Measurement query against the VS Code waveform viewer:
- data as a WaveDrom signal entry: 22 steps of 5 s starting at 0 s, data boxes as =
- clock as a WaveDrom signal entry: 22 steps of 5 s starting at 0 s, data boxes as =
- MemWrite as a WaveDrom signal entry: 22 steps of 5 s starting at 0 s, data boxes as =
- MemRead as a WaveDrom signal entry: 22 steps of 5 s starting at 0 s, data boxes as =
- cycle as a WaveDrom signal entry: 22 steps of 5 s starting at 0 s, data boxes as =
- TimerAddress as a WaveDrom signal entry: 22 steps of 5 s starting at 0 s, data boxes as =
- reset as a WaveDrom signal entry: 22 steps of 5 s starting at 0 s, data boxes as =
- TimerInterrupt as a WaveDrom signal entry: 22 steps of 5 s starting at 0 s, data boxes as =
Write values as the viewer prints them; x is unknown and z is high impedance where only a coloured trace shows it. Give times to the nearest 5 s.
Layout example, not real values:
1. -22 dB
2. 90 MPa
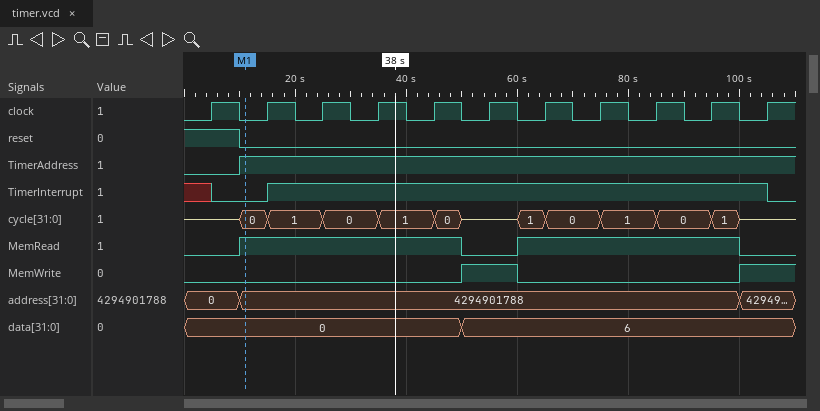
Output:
1. {name: 'data', wave: '=.........=...........', data: '0 6'}
2. {name: 'clock', wave: '0101010101010101010101'}
3. {name: 'MemWrite', wave: '0.........1.0.......1.'}
4. {name: 'MemRead', wave: '0.1.......0.1.......0.'}
5. {name: 'cycle', wave: 'z.==.=.=.=z.==.=.=.=z.', data: '0 1 0 1 0 1 0 1 0 1'}
6. {name: 'TimerAddress', wave: '0.1...................'}
7. {name: 'reset', wave: '1.0...................'}
8. {name: 'TimerInterrupt', wave: 'x0.1.................0'}
